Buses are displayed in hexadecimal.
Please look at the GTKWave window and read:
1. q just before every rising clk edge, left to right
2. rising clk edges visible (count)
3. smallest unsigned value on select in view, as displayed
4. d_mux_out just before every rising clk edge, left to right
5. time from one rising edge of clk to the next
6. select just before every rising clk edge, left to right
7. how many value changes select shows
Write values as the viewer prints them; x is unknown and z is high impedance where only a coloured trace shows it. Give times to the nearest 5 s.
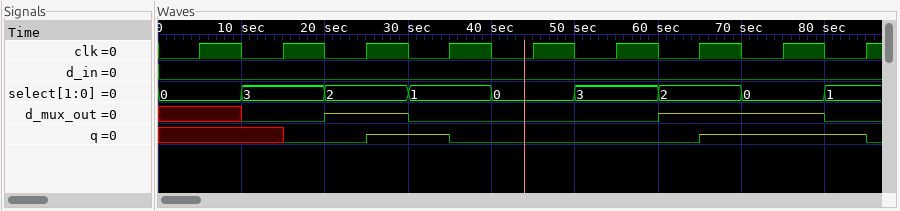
x x 0 z 0 0 0 z z
9
0
x 0 z 0 0 0 z z 0
10 s
0, 3, 2, 1, 0, 3, 2, 0, 1
8
